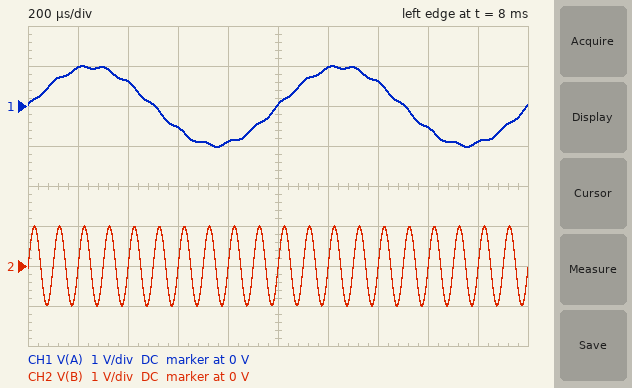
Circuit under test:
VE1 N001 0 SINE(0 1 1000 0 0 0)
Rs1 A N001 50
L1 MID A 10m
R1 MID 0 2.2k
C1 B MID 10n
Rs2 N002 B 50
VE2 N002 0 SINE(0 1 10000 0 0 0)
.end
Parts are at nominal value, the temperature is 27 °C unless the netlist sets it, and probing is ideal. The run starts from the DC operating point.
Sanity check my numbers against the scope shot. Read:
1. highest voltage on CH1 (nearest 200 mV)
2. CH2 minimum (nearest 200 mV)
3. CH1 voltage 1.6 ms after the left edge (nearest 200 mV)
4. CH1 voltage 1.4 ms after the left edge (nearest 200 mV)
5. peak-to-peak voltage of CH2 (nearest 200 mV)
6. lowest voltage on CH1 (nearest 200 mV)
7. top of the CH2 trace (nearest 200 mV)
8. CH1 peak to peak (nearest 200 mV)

1.0 V
-1.0 V
-600 mV
600 mV
2.0 V
-1.0 V
1.0 V
2.0 V
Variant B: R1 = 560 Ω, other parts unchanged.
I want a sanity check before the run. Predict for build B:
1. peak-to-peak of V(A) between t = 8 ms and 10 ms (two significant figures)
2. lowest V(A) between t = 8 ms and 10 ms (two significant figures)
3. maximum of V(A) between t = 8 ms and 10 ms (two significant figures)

1.9 V
-940 mV
930 mV
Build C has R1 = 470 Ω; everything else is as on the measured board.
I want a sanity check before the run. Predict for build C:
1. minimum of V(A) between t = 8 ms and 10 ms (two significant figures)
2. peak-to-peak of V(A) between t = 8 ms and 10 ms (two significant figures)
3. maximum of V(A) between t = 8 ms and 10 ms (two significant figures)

-920 mV
1.8 V
910 mV
